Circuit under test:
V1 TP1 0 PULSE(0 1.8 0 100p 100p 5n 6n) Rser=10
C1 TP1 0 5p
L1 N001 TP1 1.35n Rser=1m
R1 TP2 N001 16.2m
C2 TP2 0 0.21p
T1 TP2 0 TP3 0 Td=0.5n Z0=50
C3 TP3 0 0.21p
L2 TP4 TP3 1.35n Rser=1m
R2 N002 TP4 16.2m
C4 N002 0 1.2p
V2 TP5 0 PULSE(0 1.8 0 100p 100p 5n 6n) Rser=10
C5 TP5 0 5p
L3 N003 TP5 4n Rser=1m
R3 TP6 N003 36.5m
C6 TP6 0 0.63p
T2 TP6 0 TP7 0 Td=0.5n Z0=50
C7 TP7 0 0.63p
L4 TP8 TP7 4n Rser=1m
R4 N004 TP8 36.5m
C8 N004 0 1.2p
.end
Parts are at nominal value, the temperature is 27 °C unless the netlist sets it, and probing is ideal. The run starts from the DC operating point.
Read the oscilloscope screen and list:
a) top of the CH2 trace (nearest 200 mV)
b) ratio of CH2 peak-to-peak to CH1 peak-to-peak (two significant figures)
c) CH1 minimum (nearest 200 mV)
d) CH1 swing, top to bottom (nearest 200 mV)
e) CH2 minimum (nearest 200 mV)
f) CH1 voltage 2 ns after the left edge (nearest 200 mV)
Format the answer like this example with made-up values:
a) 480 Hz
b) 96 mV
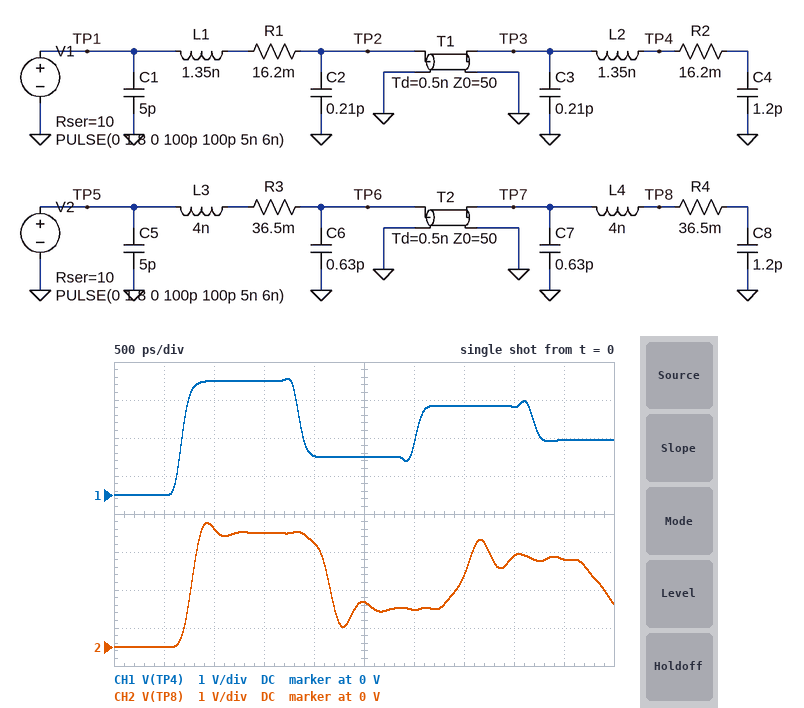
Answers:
a) 3.2 V
b) 1.1
c) 0 V
d) 3.0 V
e) 0 V
f) 1.0 V
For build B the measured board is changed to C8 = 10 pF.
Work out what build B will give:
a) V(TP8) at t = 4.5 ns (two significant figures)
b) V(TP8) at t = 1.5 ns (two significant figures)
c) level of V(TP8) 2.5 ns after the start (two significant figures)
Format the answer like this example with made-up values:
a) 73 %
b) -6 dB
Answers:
a) 980 mV
b) 2.4 V
c) 3.2 V
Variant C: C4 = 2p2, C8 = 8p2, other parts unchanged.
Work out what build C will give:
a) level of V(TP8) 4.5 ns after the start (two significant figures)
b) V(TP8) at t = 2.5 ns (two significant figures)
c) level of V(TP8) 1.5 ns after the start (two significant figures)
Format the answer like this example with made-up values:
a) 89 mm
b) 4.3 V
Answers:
a) 1.2 V
b) 3.0 V
c) 2.6 V
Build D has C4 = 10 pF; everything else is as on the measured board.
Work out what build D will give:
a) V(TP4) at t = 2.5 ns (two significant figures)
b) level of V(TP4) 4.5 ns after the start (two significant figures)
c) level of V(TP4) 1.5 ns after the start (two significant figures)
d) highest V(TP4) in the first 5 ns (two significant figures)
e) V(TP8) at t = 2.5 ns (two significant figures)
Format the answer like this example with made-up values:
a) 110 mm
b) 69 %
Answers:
a) 2.6 V
b) 1.2 V
c) 2.5 V
d) 3.2 V
e) 1.2 V
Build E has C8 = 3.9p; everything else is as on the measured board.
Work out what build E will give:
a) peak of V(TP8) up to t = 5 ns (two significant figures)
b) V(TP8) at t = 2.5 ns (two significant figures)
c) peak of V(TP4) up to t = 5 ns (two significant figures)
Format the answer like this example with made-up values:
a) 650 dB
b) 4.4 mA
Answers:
a) 3.2 V
b) 1.7 V
c) 3.1 V
